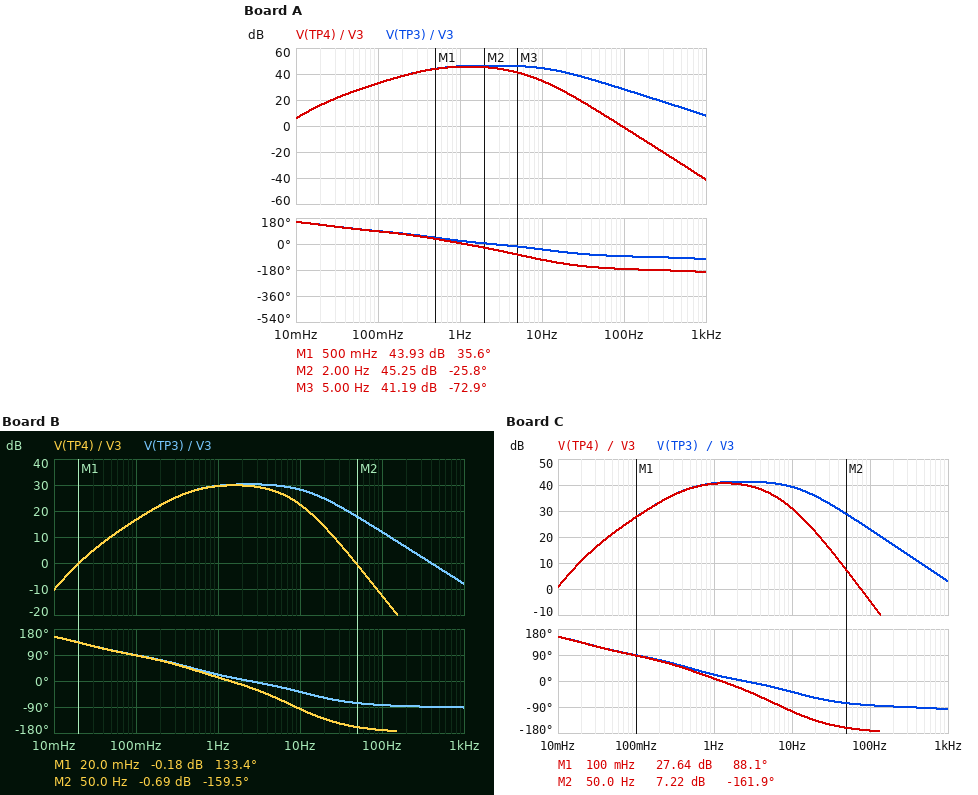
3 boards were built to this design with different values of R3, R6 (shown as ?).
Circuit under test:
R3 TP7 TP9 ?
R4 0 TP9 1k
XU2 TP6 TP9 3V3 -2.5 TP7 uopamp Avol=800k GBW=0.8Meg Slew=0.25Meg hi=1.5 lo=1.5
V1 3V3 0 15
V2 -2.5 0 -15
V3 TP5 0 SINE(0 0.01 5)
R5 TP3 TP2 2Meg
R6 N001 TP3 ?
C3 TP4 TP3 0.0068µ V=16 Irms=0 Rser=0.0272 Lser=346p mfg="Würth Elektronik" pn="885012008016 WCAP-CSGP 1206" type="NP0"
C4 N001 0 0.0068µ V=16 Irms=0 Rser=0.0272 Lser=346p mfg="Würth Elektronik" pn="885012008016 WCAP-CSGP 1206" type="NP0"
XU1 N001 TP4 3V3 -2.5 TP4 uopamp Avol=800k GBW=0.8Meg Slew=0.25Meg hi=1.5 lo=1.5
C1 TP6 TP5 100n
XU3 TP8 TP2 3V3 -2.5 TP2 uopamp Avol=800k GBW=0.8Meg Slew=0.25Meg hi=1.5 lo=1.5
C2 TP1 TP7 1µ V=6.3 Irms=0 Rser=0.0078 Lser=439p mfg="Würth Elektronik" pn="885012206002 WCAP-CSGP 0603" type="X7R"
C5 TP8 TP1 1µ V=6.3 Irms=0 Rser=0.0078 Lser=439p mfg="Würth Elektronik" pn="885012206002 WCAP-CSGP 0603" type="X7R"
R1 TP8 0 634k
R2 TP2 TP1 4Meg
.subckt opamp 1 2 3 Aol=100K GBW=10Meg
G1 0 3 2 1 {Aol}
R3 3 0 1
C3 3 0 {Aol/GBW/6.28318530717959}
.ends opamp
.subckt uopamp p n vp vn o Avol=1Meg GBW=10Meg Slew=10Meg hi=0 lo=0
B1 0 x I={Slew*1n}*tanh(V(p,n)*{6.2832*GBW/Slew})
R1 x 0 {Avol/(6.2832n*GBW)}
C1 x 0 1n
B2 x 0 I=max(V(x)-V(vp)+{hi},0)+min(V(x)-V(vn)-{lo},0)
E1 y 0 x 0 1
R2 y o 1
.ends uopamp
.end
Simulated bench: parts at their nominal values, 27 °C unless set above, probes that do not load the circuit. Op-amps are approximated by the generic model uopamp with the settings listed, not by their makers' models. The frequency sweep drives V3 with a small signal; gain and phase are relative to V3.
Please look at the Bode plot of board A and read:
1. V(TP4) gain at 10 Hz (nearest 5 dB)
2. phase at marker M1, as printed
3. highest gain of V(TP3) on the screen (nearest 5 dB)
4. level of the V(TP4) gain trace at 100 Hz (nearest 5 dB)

35 dB
35.6 deg
45 dB
0 dB
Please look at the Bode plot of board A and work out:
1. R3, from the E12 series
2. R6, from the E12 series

220 kΩ
6.8 MΩ
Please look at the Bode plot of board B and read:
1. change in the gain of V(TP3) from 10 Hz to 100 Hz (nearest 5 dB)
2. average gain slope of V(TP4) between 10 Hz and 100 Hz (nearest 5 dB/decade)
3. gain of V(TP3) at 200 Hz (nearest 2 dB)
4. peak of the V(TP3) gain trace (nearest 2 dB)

-15 dB
-35 dB/decade
6 dB
30 dB
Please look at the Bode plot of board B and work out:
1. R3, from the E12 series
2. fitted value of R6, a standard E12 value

33 kΩ
3.9 MΩ
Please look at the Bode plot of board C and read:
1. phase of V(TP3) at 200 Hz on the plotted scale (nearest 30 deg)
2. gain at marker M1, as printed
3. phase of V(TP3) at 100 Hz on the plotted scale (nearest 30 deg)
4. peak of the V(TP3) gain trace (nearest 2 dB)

-90 deg
27.64 dB
-90 deg
42 dB
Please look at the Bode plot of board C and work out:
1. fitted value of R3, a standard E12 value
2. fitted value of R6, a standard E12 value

120 kΩ
5.6 MΩ
